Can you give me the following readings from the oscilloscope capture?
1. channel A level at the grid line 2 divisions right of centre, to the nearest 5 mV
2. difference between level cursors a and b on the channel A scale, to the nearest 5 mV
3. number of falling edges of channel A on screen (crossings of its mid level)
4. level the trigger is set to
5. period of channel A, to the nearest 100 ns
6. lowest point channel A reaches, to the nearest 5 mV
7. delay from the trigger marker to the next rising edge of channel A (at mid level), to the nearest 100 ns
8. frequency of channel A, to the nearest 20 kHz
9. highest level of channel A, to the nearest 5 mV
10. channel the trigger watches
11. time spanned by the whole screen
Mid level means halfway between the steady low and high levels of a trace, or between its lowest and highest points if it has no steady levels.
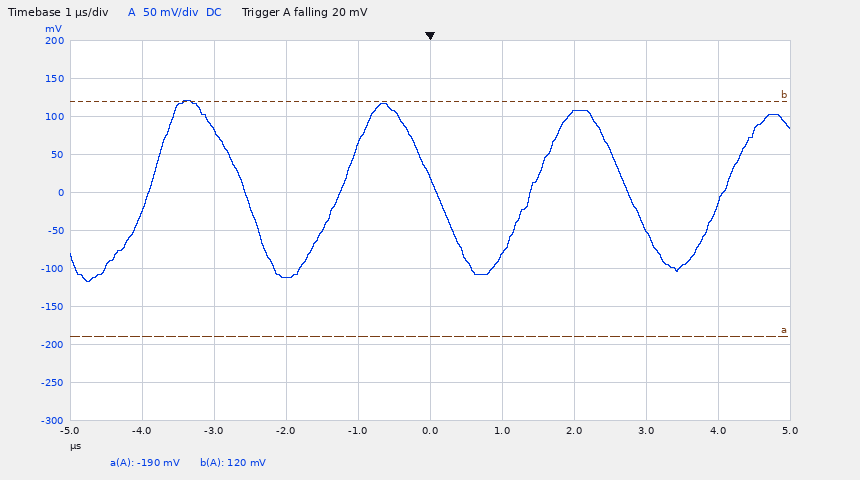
105 mV
310 mV
3
20 mV
2.7 µs
-115 mV
1.4 µs
380 kHz
120 mV
channel A
10 µs
